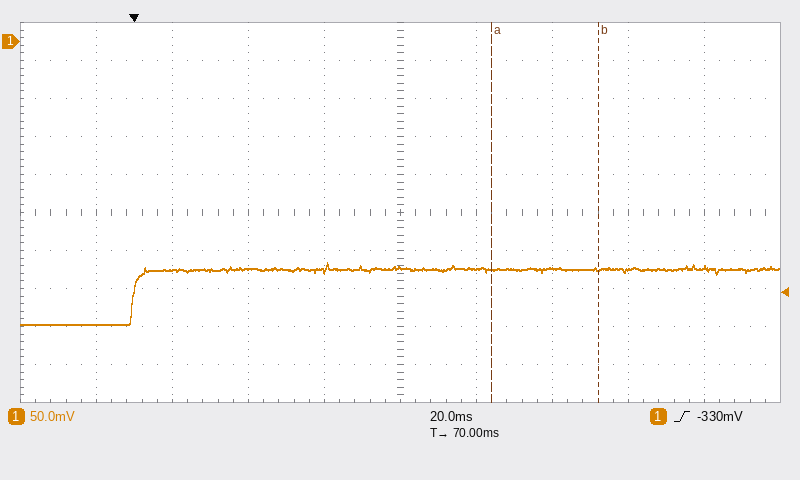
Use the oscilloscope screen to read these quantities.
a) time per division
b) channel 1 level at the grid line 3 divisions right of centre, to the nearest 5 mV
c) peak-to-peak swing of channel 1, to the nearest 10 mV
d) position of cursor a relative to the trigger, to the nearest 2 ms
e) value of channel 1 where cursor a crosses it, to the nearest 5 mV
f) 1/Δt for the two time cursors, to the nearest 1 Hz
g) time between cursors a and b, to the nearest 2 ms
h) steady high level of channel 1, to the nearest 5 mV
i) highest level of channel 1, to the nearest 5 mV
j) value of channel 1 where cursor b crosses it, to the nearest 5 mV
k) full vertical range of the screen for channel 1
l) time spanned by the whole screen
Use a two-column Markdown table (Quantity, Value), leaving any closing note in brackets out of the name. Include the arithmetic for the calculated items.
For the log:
| Quantity | Value |
|---|---|
| time per division | 20 ms |
| channel 1 level at the grid line 3 divisions right of centre, to the nearest 5 mV | -300 mV |
| peak-to-peak swing of channel 1, to the nearest 10 mV | 80 mV |
| position of cursor a relative to the trigger, to the nearest 2 ms | +94 ms |
| value of channel 1 where cursor a crosses it, to the nearest 5 mV | -300 mV |
| 1/Δt for the two time cursors, to the nearest 1 Hz | 1 / 28 ms ≈ 36 Hz |
| time between cursors a and b, to the nearest 2 ms | 28 ms |
| steady high level of channel 1, to the nearest 5 mV | -300 mV |
| highest level of channel 1, to the nearest 5 mV | -290 mV |
| value of channel 1 where cursor b crosses it, to the nearest 5 mV | -300 mV |
| full vertical range of the screen for channel 1 | 500 mV |
| time spanned by the whole screen | 200 ms |
